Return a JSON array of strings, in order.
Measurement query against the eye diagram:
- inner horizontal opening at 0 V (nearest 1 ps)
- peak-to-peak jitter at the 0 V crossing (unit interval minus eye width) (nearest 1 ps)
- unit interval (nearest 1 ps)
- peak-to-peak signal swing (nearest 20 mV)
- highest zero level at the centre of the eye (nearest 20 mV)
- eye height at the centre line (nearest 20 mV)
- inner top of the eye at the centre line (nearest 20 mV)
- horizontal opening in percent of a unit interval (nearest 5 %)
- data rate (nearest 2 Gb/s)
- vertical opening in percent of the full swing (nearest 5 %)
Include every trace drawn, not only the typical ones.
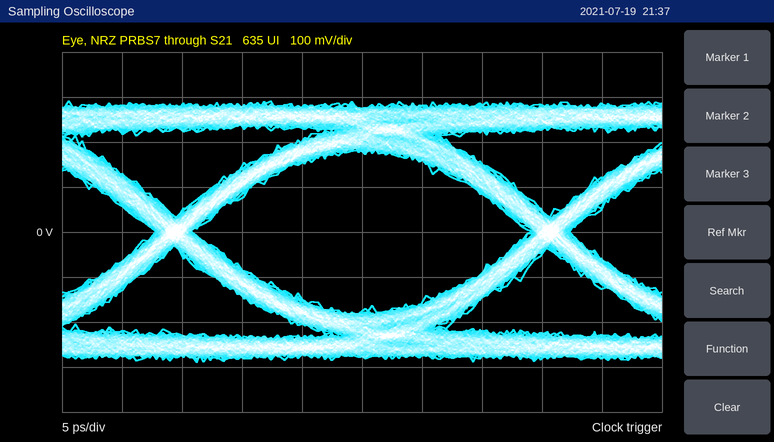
["28 ps", "3 ps", "31 ps", "580 mV", "-180 mV", "360 mV", "180 mV", "90 %", "32 Gb/s", "60 %"]
